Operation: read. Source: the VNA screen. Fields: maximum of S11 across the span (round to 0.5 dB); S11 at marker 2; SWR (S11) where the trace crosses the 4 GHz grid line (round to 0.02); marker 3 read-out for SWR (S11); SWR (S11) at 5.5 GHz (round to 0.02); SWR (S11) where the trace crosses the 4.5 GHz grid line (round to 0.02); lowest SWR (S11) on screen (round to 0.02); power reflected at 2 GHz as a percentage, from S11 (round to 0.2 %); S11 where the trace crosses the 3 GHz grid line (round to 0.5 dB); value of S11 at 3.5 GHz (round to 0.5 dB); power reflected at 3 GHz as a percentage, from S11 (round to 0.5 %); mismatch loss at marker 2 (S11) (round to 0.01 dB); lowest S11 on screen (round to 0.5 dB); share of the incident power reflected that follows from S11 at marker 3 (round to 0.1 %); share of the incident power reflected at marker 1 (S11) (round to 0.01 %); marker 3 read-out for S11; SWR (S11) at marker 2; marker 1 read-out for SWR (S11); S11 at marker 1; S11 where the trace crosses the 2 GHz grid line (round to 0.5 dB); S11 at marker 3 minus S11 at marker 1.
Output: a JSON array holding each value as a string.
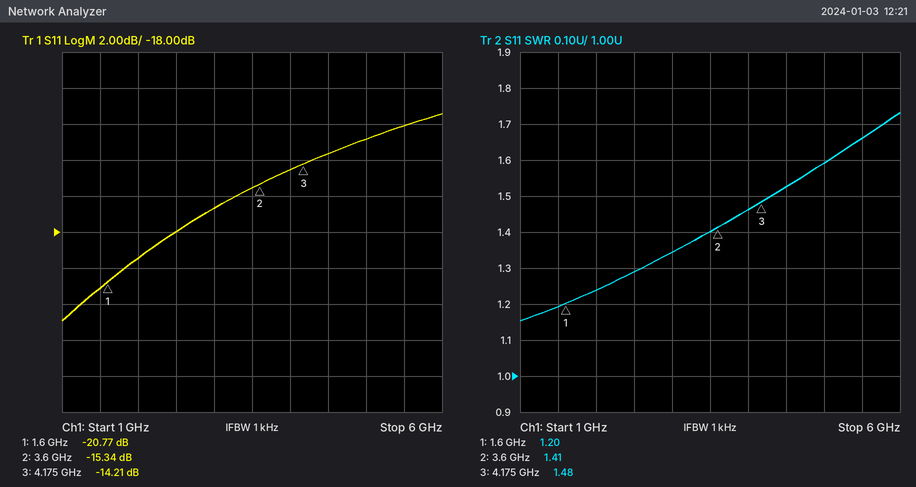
["-11.5 dB", "-15.34 dB", "1.46", "1.48", "1.66", "1.52", "1.16", "1.2 %", "-16.5 dB", "-15.5 dB", "2.0 %", "0.13 dB", "-23.0 dB", "3.8 %", "0.84 %", "-14.21 dB", "1.41", "1.20", "-20.77 dB", "-19.5 dB", "6.56 dB"]
